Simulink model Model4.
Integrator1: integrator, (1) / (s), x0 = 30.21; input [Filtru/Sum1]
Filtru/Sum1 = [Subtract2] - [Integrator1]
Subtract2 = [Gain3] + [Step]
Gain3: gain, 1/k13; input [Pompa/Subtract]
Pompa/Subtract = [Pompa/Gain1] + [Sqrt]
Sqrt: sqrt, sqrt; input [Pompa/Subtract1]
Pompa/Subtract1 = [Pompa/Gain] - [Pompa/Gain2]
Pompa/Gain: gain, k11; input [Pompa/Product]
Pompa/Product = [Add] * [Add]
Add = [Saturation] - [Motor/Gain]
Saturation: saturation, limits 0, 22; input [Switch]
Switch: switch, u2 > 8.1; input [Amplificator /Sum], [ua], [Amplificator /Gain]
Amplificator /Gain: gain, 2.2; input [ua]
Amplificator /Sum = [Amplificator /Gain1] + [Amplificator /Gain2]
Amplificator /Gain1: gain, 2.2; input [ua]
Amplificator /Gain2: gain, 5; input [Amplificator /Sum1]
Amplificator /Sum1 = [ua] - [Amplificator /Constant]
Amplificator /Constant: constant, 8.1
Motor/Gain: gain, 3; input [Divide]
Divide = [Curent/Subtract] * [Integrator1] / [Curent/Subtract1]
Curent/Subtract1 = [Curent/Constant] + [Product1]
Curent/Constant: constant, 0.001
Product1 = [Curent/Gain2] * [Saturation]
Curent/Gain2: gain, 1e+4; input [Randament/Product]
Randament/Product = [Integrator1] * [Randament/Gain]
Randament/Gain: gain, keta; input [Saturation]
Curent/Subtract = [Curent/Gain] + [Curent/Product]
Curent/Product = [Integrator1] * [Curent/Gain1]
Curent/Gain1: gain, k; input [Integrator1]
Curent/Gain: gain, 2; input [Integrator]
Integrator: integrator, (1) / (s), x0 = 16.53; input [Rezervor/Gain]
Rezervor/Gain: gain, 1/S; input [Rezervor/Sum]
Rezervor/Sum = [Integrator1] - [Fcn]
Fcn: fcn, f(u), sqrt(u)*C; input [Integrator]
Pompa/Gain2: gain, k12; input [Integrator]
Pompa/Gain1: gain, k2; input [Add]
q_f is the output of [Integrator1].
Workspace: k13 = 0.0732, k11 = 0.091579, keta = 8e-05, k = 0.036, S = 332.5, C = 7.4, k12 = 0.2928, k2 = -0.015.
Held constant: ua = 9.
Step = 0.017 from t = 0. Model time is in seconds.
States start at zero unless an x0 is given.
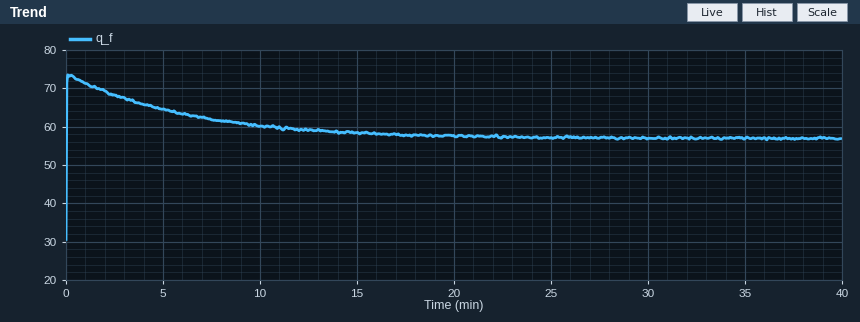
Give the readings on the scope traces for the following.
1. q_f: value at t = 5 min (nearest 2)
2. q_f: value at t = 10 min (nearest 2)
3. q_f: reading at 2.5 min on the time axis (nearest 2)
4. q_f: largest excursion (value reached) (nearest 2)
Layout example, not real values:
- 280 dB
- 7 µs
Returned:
- 64
- 60
- 68
- 74
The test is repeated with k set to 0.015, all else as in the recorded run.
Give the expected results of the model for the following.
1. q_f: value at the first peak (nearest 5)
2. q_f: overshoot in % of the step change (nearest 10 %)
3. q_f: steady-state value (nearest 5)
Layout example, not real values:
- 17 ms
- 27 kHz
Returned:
- 75
- 70 %
- 60
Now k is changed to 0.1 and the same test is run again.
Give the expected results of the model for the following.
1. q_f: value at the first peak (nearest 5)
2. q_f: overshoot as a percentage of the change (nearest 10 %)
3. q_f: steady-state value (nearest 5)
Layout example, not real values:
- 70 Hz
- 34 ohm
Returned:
- 65
- 50 %
- 55
